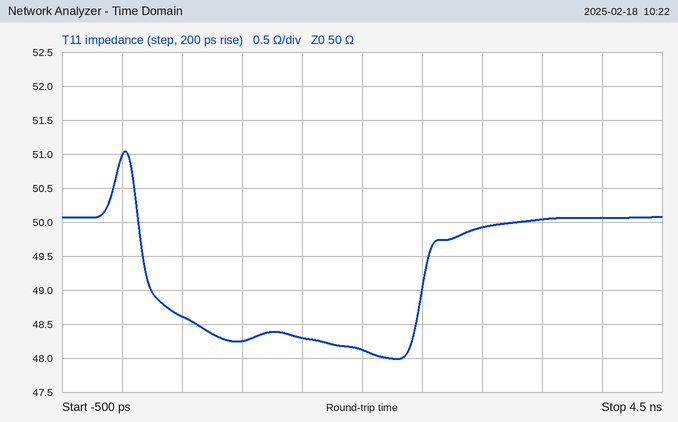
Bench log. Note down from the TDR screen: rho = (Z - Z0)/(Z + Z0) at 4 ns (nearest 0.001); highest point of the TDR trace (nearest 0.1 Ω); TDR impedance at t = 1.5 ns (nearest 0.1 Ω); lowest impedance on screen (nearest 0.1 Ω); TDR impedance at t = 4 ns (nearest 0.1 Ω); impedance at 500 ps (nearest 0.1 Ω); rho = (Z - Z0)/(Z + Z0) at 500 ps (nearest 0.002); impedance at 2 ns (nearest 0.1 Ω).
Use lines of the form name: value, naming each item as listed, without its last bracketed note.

rho = (Z - Z0)/(Z + Z0) at 4 ns: +0.001
highest point of the TDR trace: 51.0 Ω
TDR impedance at t = 1.5 ns: 48.3 Ω
lowest impedance on screen: 48.0 Ω
TDR impedance at t = 4 ns: 50.1 Ω
impedance at 500 ps: 48.6 Ω
rho = (Z - Z0)/(Z + Z0) at 500 ps: -0.014
impedance at 2 ns: 48.1 Ω
